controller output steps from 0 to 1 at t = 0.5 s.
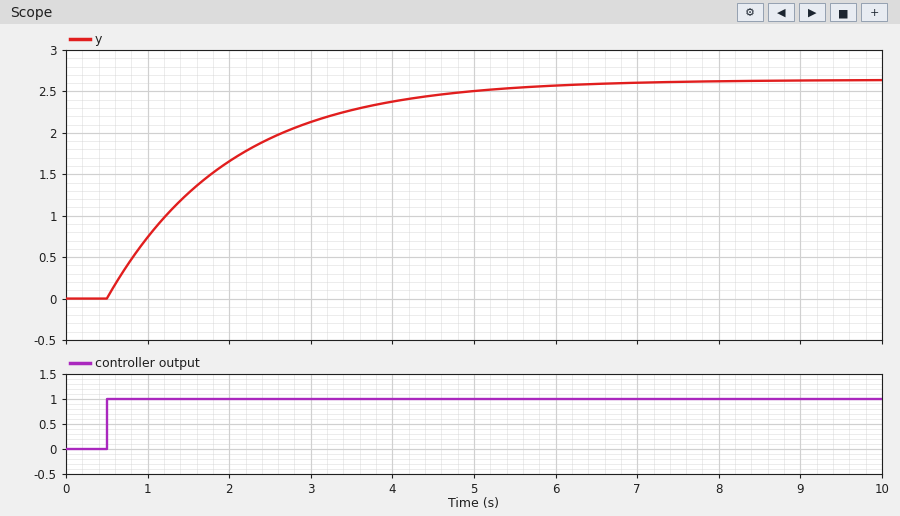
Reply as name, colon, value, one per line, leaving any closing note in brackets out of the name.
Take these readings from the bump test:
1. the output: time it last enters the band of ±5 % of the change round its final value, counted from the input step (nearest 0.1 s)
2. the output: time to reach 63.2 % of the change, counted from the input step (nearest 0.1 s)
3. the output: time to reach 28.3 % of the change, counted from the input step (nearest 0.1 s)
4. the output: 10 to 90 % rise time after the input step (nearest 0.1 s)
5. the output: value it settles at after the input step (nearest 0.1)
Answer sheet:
the output: time it last enters the band of ±5 % of the change round its final value, counted from the input step: 4.6 s
the output: time to reach 63.2 % of the change, counted from the input step: 1.5 s
the output: time to reach 28.3 % of the change, counted from the input step: 0.5 s
the output: 10 to 90 % rise time after the input step: 3.3 s
the output: value it settles at after the input step: 2.6
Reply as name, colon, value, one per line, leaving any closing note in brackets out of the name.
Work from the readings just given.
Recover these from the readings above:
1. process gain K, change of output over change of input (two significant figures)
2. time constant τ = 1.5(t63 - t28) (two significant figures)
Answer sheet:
process gain K, change of output over change of input: 2.6
time constant τ = 1.5(t63 - t28): 1.5 s
